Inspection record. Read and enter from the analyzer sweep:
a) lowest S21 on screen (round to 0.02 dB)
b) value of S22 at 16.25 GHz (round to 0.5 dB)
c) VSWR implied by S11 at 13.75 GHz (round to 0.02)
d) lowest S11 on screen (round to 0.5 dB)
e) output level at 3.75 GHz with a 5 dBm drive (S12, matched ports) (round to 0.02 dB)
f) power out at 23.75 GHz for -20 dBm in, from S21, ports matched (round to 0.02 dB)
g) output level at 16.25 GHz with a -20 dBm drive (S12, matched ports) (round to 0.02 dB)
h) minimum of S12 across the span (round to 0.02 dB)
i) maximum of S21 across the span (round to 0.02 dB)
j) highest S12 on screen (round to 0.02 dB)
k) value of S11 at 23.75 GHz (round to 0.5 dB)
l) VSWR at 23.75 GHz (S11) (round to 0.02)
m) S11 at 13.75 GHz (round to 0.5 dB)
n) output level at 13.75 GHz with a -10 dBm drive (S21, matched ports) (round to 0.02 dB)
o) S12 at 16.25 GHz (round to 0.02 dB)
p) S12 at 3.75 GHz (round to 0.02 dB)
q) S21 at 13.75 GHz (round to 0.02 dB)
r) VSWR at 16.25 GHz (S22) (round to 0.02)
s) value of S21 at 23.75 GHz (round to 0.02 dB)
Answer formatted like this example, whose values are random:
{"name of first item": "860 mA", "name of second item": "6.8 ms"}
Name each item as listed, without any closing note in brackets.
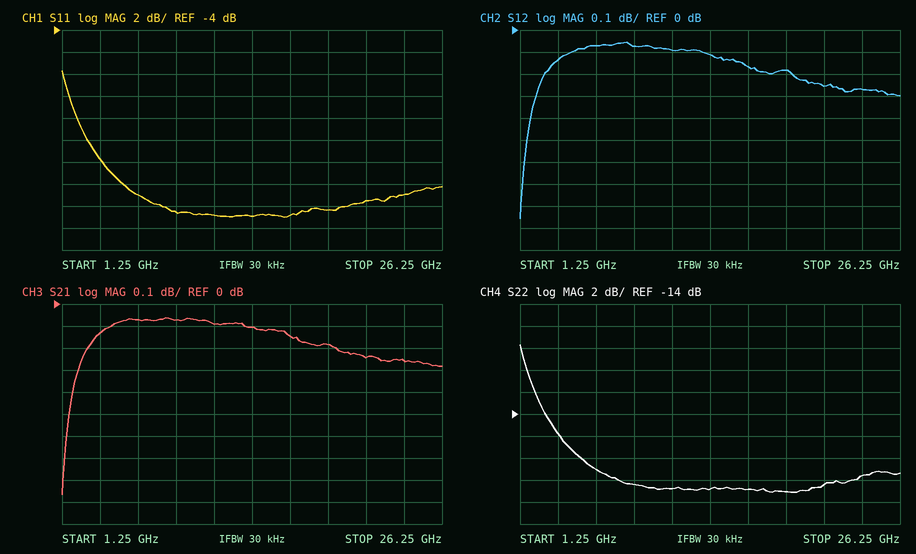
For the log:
{"lowest S21 on screen": "-0.86 dB", "value of S22 at 16.25 GHz": "-21.0 dB", "VSWR implied by S11 at 13.75 GHz": "1.20", "lowest S11 on screen": "-21.0 dB", "output level at 3.75 GHz with a 5 dBm drive (S12, matched ports)": "4.86 dBm", "power out at 23.75 GHz for -20 dBm in, from S21, ports matched": "-20.26 dBm", "output level at 16.25 GHz with a -20 dBm drive (S12, matched ports)": "-20.16 dBm", "minimum of S12 across the span": "-0.86 dB", "maximum of S21 across the span": "-0.06 dB", "highest S12 on screen": "-0.06 dB", "value of S11 at 23.75 GHz": "-19.0 dB", "VSWR at 23.75 GHz (S11)": "1.26", "S11 at 13.75 GHz": "-21.0 dB", "output level at 13.75 GHz with a -10 dBm drive (S21, matched ports)": "-10.10 dBm", "S12 at 16.25 GHz": "-0.16 dB", "S12 at 3.75 GHz": "-0.14 dB", "S21 at 13.75 GHz": "-0.10 dB", "VSWR at 16.25 GHz (S22)": "1.20", "value of S21 at 23.75 GHz": "-0.26 dB"}
